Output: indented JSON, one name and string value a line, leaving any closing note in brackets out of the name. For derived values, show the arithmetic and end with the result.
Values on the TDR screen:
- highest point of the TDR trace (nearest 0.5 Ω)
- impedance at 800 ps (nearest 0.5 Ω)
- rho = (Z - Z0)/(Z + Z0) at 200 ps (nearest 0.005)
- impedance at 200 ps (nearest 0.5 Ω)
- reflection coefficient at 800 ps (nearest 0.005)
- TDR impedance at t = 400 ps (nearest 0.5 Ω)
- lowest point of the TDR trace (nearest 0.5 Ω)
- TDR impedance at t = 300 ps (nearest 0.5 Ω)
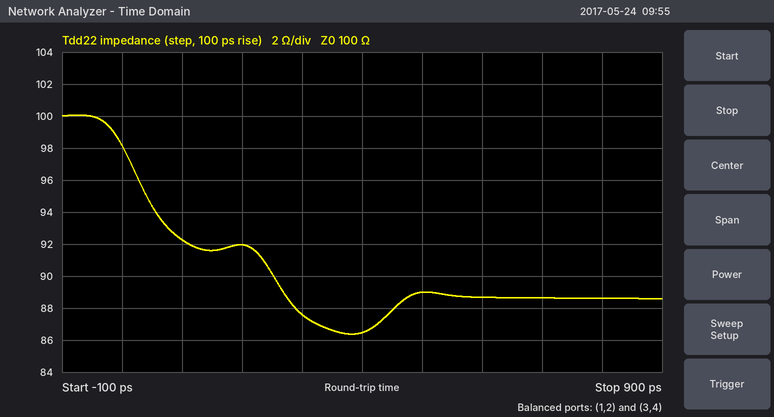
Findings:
{
  "highest point of the TDR trace": "100.0 Ω",
  "impedance at 800 ps": "88.5 Ω",
  "rho = (Z - Z0)/(Z + Z0) at 200 ps": "(92 − 100)/(92 + 100) ≈ -0.0417, so -0.040 to the nearest 0.005",
  "impedance at 200 ps": "92.0 Ω",
  "reflection coefficient at 800 ps": "(88.5 − 100)/(88.5 + 100) ≈ -0.0610, so -0.060 to the nearest 0.005",
  "TDR impedance at t = 400 ps": "86.5 Ω",
  "lowest point of the TDR trace": "86.5 Ω",
  "TDR impedance at t = 300 ps": "87.5 Ω"
}
